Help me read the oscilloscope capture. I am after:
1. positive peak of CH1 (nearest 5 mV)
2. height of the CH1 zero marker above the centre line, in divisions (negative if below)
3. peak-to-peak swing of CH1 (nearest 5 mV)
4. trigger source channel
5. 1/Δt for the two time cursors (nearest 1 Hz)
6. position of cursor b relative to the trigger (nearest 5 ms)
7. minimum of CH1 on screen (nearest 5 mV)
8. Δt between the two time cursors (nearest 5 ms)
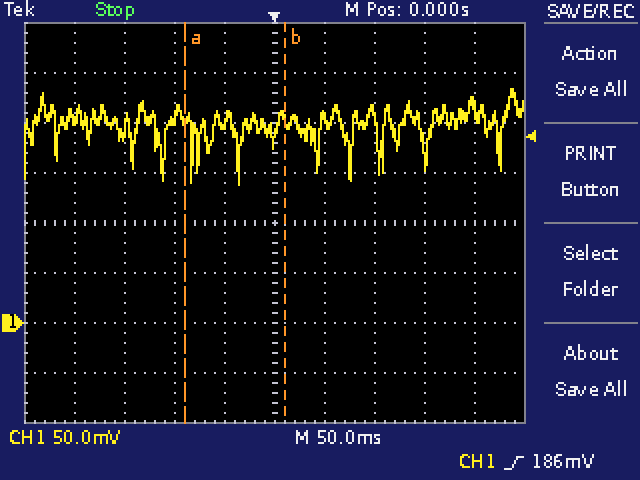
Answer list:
235 mV
-2.0 div
95 mV
CH1
10 Hz
+10 ms
140 mV
100 ms
